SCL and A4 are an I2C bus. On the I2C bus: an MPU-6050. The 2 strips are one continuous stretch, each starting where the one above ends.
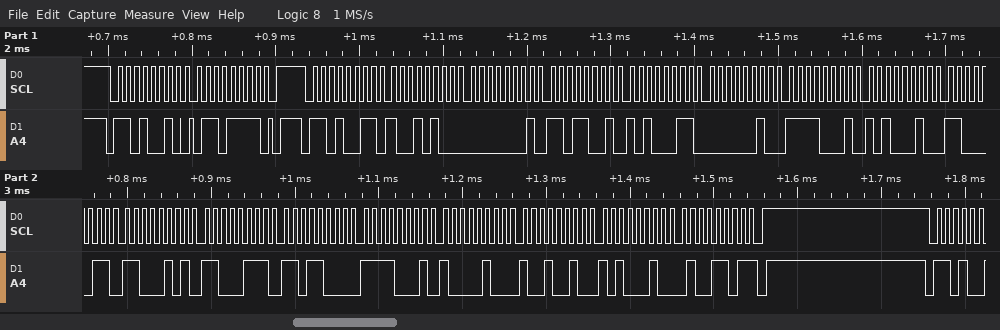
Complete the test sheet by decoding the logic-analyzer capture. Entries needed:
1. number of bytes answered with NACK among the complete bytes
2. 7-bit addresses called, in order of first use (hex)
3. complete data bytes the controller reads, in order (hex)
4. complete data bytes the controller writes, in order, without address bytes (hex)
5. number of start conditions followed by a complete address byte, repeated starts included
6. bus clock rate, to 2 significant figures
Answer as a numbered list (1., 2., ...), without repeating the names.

1. 1
2. 0x69
3. 94 01 D9 A3 02 F1 A2 C3 C5 C7 D8 F1 84 92 A2 4D
4. 6F
5. 2
6. 100 kHz
